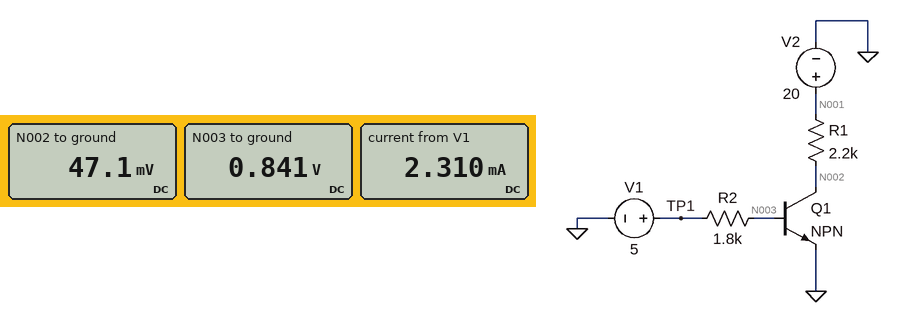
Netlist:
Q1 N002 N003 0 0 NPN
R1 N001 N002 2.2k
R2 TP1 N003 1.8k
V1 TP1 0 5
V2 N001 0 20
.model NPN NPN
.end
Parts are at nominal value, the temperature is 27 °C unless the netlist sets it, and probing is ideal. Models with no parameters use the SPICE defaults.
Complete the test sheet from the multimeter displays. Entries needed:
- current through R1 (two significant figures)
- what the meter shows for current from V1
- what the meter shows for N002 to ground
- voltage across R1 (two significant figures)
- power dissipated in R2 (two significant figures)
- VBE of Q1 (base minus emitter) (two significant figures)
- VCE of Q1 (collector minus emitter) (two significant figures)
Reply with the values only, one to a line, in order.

9.1 mA
2.310 mA
47.1 mV
20 V
9.6 mW
840 mV
47 mV
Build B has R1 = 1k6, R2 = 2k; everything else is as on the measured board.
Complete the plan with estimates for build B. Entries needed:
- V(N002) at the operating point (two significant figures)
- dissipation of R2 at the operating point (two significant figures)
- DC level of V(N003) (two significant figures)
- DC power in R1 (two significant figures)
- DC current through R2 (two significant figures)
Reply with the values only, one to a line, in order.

55 mV
8.6 mW
850 mV
250 mW
2.1 mA
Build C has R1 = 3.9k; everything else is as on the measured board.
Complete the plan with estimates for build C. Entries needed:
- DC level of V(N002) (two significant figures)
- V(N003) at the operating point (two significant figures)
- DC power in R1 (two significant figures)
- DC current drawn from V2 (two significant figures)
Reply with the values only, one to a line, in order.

38 mV
830 mV
100 mW
5.1 mA
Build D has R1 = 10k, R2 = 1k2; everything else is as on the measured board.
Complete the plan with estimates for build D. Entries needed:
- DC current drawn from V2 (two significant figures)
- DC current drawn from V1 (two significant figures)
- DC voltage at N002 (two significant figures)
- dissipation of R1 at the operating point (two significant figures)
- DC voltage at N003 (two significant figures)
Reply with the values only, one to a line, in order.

2.0 mA
3.5 mA
25 mV
40 mW
830 mV
